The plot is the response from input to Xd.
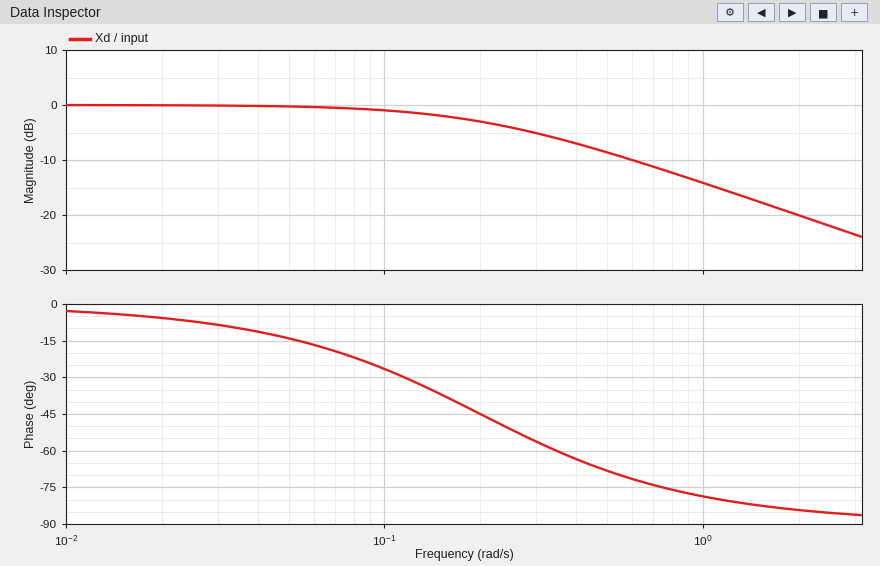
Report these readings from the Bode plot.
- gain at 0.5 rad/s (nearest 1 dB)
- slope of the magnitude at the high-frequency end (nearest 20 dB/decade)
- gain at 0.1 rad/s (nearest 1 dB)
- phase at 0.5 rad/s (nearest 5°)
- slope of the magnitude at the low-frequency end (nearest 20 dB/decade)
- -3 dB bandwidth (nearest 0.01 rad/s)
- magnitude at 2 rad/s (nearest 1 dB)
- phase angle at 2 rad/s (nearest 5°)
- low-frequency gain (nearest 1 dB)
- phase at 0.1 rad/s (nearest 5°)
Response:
-9 dB
-20 dB/decade
-1 dB
-70°
0 dB/decade
0.20 rad/s
-20 dB
-85°
0 dB
-25°
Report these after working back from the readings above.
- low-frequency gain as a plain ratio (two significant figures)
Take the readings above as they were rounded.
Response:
1.0
